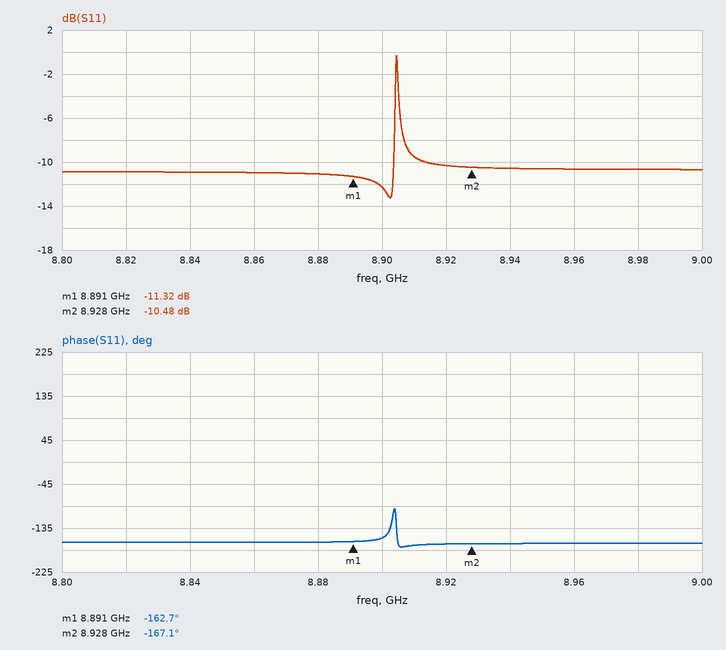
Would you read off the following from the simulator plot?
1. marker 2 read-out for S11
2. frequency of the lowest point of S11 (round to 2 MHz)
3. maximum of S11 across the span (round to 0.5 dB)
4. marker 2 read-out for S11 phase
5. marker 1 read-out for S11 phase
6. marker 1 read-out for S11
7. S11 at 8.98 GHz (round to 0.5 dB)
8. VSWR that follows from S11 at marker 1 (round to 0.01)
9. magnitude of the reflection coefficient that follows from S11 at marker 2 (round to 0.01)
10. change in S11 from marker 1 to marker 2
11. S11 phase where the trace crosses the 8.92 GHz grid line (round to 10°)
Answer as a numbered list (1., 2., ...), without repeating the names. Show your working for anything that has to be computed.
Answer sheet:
1. -10.48 dB
2. 8.902 GHz
3. -0.5 dB
4. -167.1°
5. -162.7°
6. -11.32 dB
7. -10.5 dB
8. (1 + 0.2716)/(1 − 0.2716) ≈ 1.75
9. 10^(-10.48/20) ≈ 0.30
10. -10.48 − (-11.32) = 0.84 dB
11. -170°
